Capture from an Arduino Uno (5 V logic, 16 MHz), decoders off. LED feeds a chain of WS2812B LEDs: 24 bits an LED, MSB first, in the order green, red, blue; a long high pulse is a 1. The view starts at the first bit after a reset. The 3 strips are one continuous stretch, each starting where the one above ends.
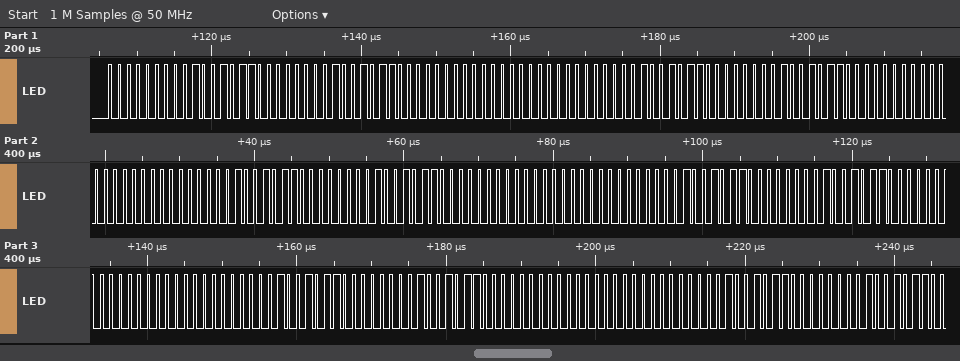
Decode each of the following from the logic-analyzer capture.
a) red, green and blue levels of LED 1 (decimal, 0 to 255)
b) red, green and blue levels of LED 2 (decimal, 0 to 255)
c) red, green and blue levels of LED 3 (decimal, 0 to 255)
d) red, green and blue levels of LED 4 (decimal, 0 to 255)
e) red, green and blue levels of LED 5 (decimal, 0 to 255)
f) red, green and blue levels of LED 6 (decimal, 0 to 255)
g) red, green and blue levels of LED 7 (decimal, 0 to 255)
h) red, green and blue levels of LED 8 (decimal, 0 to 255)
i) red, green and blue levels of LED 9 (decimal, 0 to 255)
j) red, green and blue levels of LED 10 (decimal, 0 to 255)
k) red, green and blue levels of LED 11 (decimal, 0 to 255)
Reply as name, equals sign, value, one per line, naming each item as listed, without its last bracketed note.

red, green and blue levels of LED 1 = 75, 0, 0
red, green and blue levels of LED 2 = 0, 150, 0
red, green and blue levels of LED 3 = 75, 0, 0
red, green and blue levels of LED 4 = 0, 150, 0
red, green and blue levels of LED 5 = 75, 0, 0
red, green and blue levels of LED 6 = 0, 150, 0
red, green and blue levels of LED 7 = 75, 0, 0
red, green and blue levels of LED 8 = 0, 150, 0
red, green and blue levels of LED 9 = 75, 0, 0
red, green and blue levels of LED 10 = 0, 150, 0
red, green and blue levels of LED 11 = 75, 0, 0
